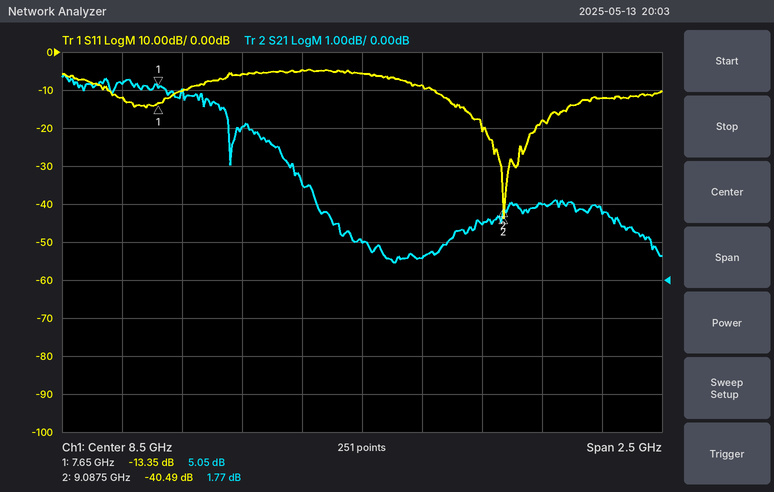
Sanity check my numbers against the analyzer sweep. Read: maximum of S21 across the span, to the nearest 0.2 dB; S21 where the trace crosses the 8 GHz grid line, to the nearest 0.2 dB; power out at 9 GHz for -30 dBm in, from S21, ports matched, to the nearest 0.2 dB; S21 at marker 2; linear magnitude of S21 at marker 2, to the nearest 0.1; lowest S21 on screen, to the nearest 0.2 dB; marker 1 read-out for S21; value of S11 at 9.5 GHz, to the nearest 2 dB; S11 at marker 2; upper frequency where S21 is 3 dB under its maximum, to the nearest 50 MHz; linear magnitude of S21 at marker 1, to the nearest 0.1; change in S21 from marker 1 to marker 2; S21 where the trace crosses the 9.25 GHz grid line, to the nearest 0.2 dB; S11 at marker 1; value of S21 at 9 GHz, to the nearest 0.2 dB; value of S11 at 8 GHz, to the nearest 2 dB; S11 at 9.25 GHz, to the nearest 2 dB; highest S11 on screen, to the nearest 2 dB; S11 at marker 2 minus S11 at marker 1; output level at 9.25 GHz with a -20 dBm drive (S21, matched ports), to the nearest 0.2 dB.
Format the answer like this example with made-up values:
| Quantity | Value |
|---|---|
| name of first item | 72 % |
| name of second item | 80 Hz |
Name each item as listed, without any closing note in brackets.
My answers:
| Quantity | Value |
|---|---|
| maximum of S21 across the span, to the nearest 0.2 dB | 5.4 dB |
| S21 where the trace crosses the 8 GHz grid line, to the nearest 0.2 dB | 4.0 dB |
| power out at 9 GHz for -30 dBm in, from S21, ports matched, to the nearest 0.2 dB | -28.6 dBm |
| S21 at marker 2 | 1.77 dB |
| linear magnitude of S21 at marker 2, to the nearest 0.1 | 1.2 |
| lowest S21 on screen, to the nearest 0.2 dB | 0.4 dB |
| marker 1 read-out for S21 | 5.05 dB |
| value of S11 at 9.5 GHz, to the nearest 2 dB | -12 dB |
| S11 at marker 2 | -40.49 dB |
| upper frequency where S21 is 3 dB under its maximum, to the nearest 50 MHz | 8.30 GHz |
| linear magnitude of S21 at marker 1, to the nearest 0.1 | 1.8 |
| change in S21 from marker 1 to marker 2 | -3.28 dB |
| S21 where the trace crosses the 9.25 GHz grid line, to the nearest 0.2 dB | 2.0 dB |
| S11 at marker 1 | -13.35 dB |
| value of S21 at 9 GHz, to the nearest 0.2 dB | 1.4 dB |
| value of S11 at 8 GHz, to the nearest 2 dB | -6 dB |
| S11 at 9.25 GHz, to the nearest 2 dB | -18 dB |
| highest S11 on screen, to the nearest 2 dB | -4 dB |
| S11 at marker 2 minus S11 at marker 1 | -27.14 dB |
| output level at 9.25 GHz with a -20 dBm drive (S21, matched ports), to the nearest 0.2 dB | -18.0 dBm |
